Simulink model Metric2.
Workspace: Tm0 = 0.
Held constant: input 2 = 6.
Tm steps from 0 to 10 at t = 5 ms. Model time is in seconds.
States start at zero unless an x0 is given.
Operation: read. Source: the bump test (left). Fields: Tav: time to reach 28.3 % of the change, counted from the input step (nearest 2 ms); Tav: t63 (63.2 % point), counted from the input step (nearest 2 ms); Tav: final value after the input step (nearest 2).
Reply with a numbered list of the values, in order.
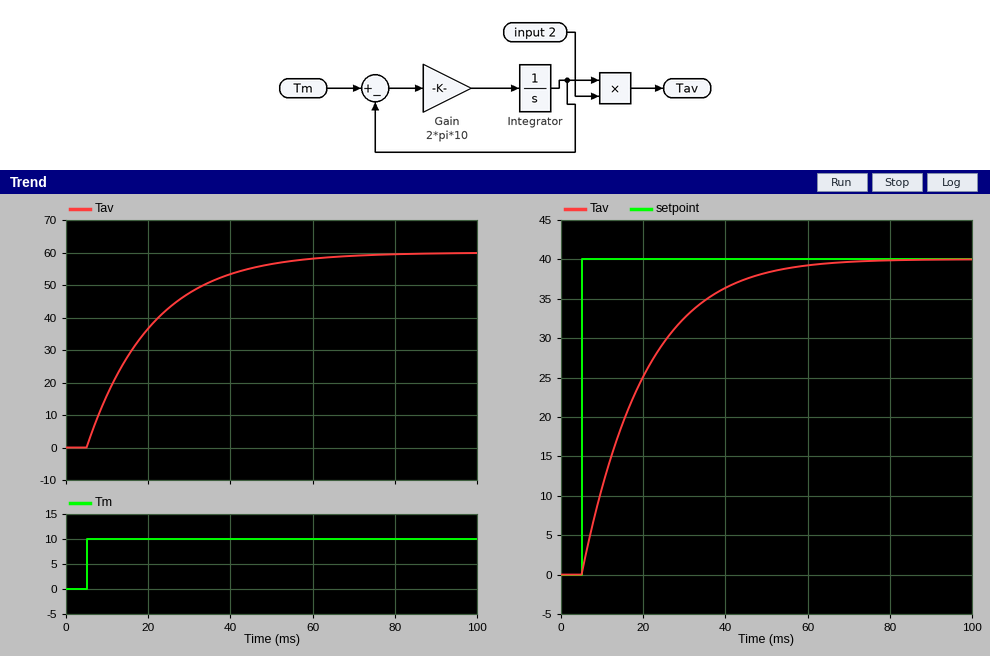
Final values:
1. 6 ms
2. 16 ms
3. 60
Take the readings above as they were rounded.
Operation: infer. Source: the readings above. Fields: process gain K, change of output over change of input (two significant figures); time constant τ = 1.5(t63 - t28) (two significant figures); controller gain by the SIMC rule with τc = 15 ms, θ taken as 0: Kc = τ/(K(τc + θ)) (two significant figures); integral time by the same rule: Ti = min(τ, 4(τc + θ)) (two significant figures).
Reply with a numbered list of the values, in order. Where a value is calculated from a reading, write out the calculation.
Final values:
1. (60 - 0) / 10 = 6.0
2. 1.5 × (16 - 6) = 15 ms
3. 15 / (6 × (15 + 0)) = 0.17
4. min(15, 4 × (15 + 0)) = 15 ms
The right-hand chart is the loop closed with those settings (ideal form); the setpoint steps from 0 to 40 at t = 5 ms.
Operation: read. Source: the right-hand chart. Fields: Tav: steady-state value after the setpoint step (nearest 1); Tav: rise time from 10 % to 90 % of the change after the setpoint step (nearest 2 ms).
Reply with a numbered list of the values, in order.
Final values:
1. 40
2. 32 ms
